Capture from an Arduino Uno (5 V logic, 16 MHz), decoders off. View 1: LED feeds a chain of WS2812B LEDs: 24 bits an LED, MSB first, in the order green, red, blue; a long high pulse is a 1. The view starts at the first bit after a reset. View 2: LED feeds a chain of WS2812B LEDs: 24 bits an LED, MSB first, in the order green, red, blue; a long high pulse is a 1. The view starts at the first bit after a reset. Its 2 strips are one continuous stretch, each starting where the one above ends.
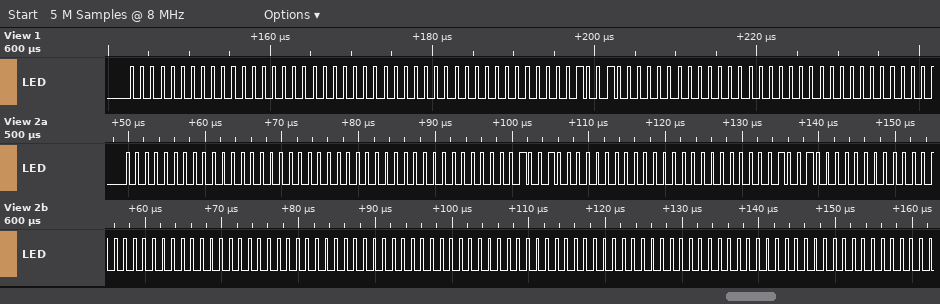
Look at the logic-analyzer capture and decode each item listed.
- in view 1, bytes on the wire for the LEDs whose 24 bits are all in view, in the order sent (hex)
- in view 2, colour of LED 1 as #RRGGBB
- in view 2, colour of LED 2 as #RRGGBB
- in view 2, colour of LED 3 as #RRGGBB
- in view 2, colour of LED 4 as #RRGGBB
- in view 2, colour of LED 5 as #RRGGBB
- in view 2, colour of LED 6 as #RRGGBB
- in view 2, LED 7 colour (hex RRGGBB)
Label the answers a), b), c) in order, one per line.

a) 00 00 00 00 00 09 00 00 00
b) #000000
c) #000048
d) #000009
e) #000000
f) #000000
g) #000000
h) #000000
